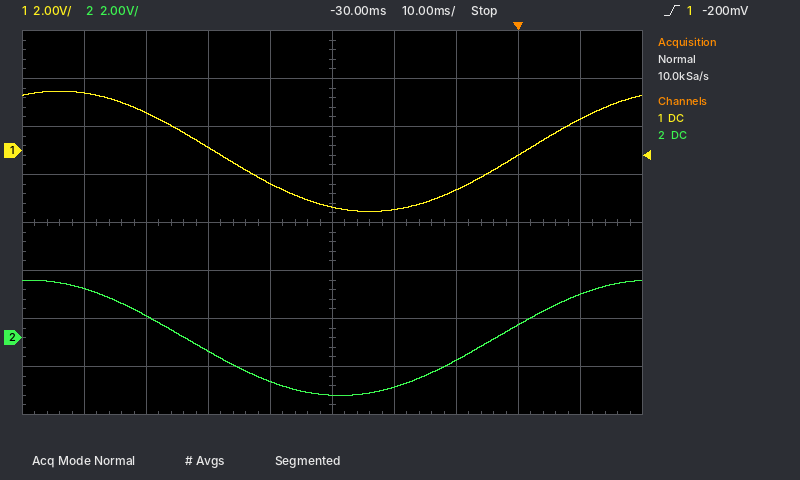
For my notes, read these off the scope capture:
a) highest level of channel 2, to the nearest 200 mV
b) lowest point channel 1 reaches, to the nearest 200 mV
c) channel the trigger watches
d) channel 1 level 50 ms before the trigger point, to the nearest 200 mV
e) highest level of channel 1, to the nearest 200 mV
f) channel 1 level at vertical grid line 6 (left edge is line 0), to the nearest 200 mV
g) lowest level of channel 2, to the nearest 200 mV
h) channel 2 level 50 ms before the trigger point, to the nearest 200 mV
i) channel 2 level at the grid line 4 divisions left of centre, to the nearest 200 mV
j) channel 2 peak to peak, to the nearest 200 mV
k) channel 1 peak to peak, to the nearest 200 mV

2.4 V
-2.6 V
channel 1
200 mV
2.4 V
-2.4 V
-2.4 V
-600 mV
2.0 V
4.8 V
5.0 V
